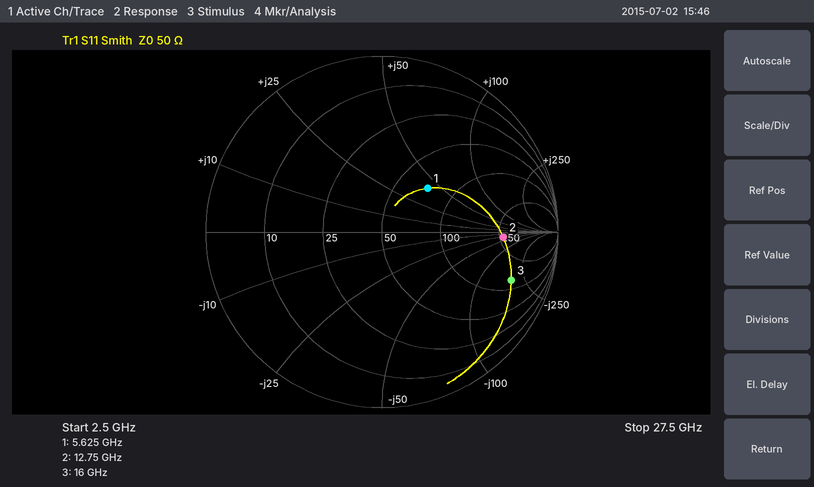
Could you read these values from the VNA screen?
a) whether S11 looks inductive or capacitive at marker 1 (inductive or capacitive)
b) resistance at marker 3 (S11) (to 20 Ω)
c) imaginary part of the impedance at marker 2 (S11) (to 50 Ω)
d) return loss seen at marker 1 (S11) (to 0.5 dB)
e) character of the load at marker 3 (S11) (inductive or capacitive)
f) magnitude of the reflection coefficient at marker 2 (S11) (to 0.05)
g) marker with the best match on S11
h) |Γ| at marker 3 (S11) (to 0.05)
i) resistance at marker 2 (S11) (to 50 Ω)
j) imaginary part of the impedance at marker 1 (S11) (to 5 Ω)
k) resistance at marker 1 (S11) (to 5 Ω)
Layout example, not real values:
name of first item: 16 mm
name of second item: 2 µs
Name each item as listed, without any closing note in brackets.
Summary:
whether S11 looks inductive or capacitive at marker 1: inductive
resistance at marker 3 (S11): 140 Ω
imaginary part of the impedance at marker 2 (S11): -50 Ω
return loss seen at marker 1 (S11): 9.0 dB
character of the load at marker 3 (S11): capacitive
magnitude of the reflection coefficient at marker 2 (S11): 0.70
marker with the best match on S11: marker 1
|Γ| at marker 3 (S11): 0.80
resistance at marker 2 (S11): 250 Ω
imaginary part of the impedance at marker 1 (S11): +40 Ω
resistance at marker 1 (S11): 70 Ω
